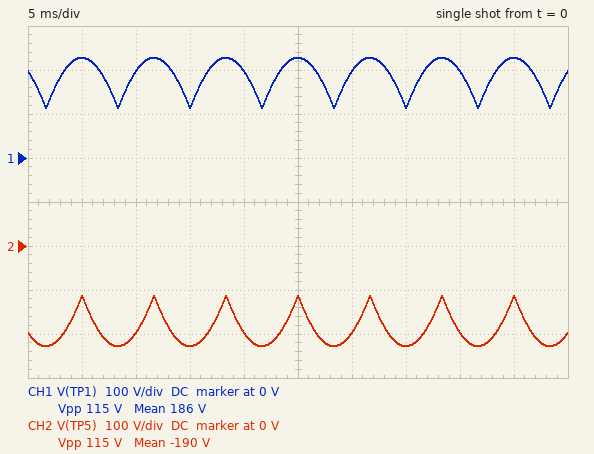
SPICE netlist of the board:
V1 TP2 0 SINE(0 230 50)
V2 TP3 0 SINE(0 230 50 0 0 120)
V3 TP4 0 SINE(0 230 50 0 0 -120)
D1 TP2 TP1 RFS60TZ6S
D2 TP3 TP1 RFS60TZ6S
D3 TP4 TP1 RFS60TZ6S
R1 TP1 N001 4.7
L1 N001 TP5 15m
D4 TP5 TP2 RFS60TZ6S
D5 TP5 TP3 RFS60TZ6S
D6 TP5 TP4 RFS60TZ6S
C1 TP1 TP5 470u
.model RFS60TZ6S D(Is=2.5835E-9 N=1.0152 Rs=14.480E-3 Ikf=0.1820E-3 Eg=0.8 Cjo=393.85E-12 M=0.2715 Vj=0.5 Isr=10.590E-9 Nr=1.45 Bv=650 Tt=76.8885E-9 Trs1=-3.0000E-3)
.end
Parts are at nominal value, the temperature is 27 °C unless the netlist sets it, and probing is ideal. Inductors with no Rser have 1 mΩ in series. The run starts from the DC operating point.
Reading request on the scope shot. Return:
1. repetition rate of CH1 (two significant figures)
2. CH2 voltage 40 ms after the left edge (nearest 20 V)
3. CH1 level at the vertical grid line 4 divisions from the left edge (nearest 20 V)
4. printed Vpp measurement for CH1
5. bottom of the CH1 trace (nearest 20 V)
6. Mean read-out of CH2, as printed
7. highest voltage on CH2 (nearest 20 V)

150 Hz
-200 V
200 V
115 V
120 V
-190 V
-120 V
